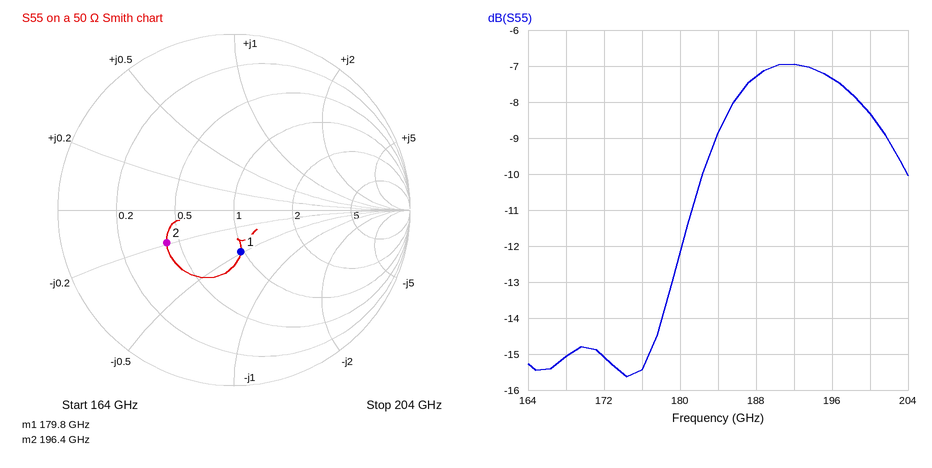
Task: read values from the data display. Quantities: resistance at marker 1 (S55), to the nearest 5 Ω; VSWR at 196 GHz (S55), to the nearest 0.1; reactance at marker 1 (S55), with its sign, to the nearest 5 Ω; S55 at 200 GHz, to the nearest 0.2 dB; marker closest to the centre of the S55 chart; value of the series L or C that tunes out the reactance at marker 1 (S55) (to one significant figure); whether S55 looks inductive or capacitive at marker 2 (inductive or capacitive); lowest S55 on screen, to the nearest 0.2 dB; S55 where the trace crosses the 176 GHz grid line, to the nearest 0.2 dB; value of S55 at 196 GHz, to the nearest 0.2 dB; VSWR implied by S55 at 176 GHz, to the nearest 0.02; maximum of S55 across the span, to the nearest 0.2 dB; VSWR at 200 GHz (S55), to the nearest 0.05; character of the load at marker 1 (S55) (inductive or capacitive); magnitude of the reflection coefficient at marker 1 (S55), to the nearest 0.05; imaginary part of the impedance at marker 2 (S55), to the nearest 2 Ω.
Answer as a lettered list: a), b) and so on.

a) 50 Ω
b) 2.5
c) -25 Ω
d) -8.4 dB
e) marker 1
f) 20 pH
g) capacitive
h) -15.6 dB
i) -15.4 dB
j) -7.4 dB
k) 1.40
l) -7.0 dB
m) 2.25
n) capacitive
o) 0.25
p) -10 Ω
